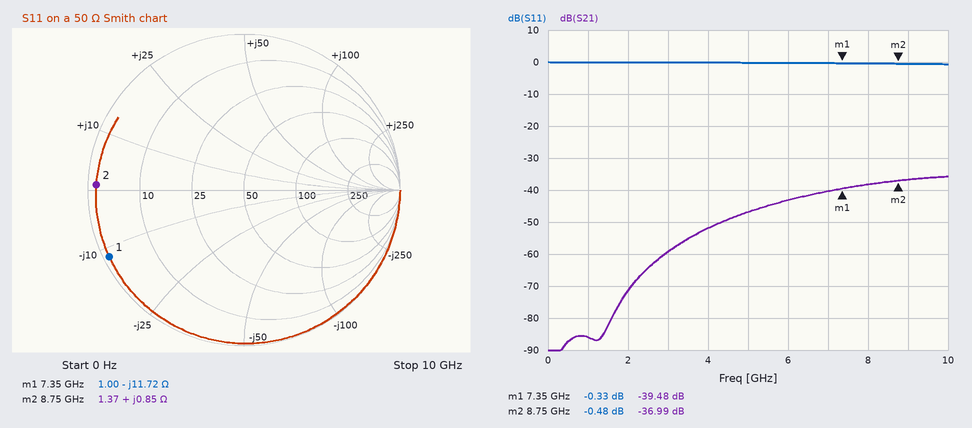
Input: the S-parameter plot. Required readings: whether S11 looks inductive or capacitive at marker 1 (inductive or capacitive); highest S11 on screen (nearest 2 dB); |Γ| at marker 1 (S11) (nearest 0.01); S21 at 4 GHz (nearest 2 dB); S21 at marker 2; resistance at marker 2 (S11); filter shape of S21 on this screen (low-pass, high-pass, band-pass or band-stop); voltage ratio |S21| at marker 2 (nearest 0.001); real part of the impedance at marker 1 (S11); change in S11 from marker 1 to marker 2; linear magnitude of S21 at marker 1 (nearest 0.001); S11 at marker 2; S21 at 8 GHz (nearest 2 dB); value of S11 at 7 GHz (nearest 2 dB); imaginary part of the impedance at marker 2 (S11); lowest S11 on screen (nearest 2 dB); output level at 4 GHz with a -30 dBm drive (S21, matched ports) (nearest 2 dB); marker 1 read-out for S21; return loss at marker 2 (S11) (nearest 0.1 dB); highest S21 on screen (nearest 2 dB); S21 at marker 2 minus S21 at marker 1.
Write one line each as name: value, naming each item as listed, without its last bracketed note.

whether S11 looks inductive or capacitive at marker 1: capacitive
highest S11 on screen: 0 dB
|Γ| at marker 1 (S11): 0.96
S21 at 4 GHz: -52 dB
S21 at marker 2: -36.99 dB
resistance at marker 2: 1.37 Ω
filter shape of S21 on this screen: high-pass
voltage ratio |S21| at marker 2: 0.014
real part of the impedance at marker 1: 1.00 Ω
change in S11 from marker 1 to marker 2: -0.15 dB
linear magnitude of S21 at marker 1: 0.011
S11 at marker 2: -0.48 dB
S21 at 8 GHz: -38 dB
value of S11 at 7 GHz: 0 dB
imaginary part of the impedance at marker 2: +0.85 Ω
lowest S11 on screen: 0 dB
output level at 4 GHz with a -30 dBm drive (S21, matched ports): -82 dBm
marker 1 read-out for S21: -39.48 dB
return loss at marker 2 (S11): 0.5 dB
highest S21 on screen: -36 dB
S21 at marker 2 minus S21 at marker 1: 2.49 dB
